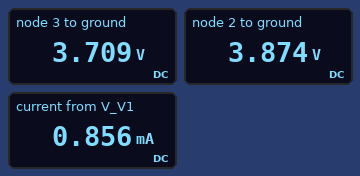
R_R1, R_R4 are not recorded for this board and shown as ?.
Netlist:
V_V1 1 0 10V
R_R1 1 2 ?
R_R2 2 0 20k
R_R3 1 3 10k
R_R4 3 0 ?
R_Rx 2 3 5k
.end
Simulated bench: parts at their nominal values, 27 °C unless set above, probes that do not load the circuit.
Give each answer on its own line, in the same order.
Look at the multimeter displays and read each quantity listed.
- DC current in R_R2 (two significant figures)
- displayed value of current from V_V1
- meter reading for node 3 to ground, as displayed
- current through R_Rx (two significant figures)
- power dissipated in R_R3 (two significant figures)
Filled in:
190 µA
0.856 mA
3.709 V
33 µA
4.0 mW
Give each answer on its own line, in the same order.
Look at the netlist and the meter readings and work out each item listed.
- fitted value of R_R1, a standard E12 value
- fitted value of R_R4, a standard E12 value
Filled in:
27 kΩ
5.6 kΩ
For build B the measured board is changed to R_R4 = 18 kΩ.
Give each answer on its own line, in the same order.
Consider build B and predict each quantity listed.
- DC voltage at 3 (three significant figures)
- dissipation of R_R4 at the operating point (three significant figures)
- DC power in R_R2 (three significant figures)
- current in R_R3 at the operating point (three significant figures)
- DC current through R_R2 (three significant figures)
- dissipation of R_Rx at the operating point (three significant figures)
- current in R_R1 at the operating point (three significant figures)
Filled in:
5.82 V
1.88 mW
1.43 mW
418 µA
267 µA
45.0 µW
172 µA
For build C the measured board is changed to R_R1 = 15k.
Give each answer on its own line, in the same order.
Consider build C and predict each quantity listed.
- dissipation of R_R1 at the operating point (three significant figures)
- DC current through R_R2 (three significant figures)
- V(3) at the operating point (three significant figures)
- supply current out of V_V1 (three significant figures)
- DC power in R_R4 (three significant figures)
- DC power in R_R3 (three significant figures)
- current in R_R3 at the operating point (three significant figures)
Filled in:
1.91 mW
233 µA
4.03 V
953 µA
2.91 mW
3.56 mW
597 µA
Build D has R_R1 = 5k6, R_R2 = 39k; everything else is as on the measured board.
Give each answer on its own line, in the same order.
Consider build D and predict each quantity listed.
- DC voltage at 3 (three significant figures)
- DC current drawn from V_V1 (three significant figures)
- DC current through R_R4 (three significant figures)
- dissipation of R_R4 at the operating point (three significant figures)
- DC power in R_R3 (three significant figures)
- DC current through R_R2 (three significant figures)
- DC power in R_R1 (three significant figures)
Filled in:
4.96 V
1.06 mA
886 µA
4.40 mW
2.54 mW
176 µA
1.75 mW
